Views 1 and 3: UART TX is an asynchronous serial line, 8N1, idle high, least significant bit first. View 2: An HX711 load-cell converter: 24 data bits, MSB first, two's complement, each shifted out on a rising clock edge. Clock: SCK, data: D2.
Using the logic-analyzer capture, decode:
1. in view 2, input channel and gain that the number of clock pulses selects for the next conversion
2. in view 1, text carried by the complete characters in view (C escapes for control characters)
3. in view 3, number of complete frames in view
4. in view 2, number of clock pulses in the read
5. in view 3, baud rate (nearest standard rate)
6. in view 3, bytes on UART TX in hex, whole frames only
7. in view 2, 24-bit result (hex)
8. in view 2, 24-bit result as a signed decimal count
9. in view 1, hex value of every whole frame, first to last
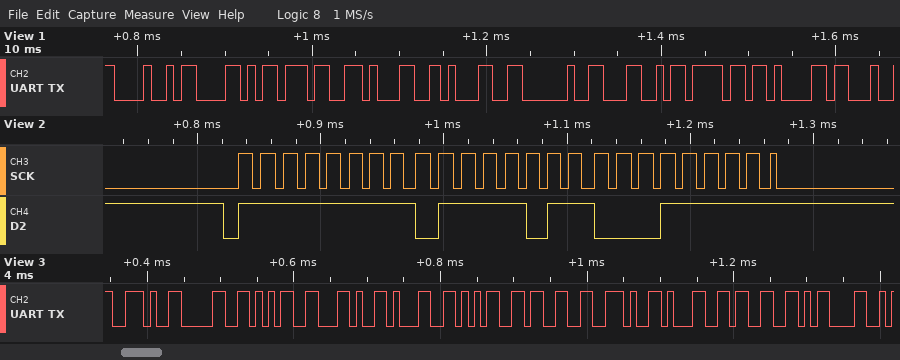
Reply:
channel A, gain 128
"HX711 Loa"
11
25
115200 baud
2E 30 35 2C 31 35 33 2E 31 33 0D
0xFF7B1F
-34017
48 58 37 31 31 20 4C 6F 61
